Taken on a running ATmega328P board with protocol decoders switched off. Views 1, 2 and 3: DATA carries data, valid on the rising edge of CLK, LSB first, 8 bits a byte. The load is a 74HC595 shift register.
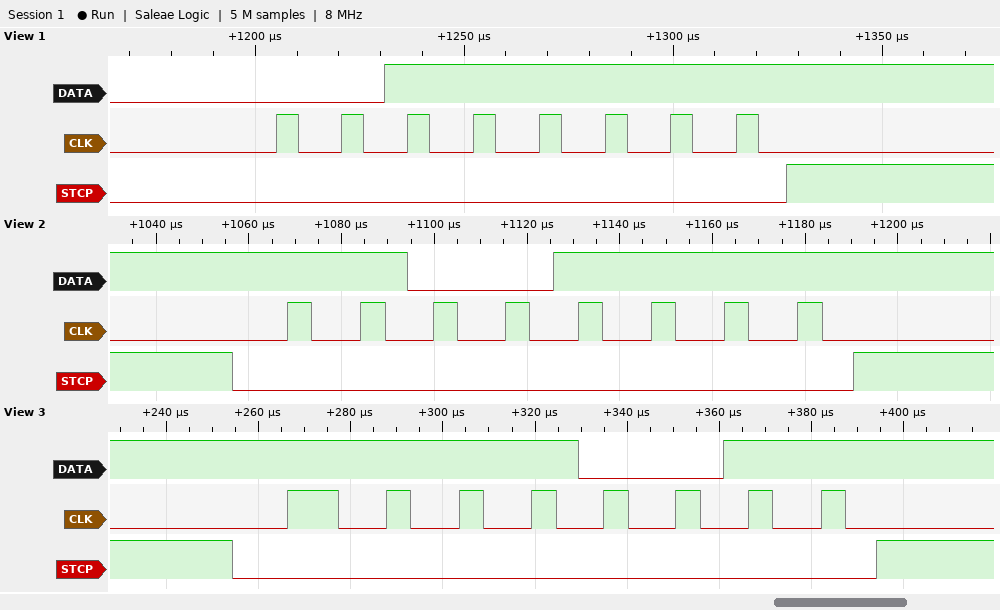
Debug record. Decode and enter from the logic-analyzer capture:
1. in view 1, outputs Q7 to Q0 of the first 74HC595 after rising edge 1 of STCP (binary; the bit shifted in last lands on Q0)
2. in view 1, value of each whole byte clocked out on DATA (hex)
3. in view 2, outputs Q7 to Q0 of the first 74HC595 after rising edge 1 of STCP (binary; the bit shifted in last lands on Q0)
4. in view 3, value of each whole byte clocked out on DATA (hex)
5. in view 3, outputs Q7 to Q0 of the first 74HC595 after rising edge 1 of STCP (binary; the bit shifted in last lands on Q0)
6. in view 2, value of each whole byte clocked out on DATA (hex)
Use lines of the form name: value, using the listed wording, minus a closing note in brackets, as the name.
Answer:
in view 1, outputs Q7 to Q0 of the first 74HC595 after rising edge 1 of STCP: 00111111
in view 1, value of each whole byte clocked out on DATA: 0xFC
in view 2, outputs Q7 to Q0 of the first 74HC595 after rising edge 1 of STCP: 11001111
in view 3, value of each whole byte clocked out on DATA: CF
in view 3, outputs Q7 to Q0 of the first 74HC595 after rising edge 1 of STCP: 11110011
in view 2, value of each whole byte clocked out on DATA: F3
